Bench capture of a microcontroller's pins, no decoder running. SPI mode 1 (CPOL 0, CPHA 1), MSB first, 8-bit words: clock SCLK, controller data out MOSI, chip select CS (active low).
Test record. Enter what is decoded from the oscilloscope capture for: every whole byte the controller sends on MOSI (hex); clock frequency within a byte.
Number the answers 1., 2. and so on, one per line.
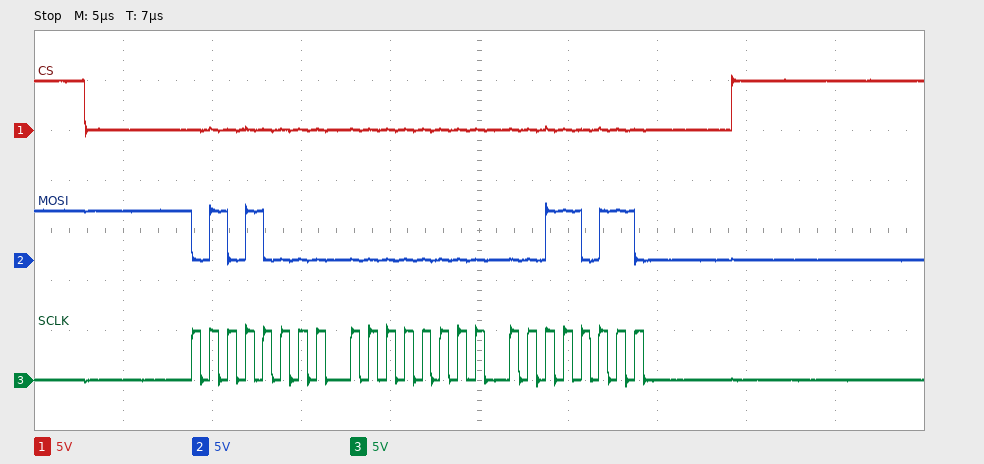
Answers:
1. 50 00 36
2. 1 MHz
